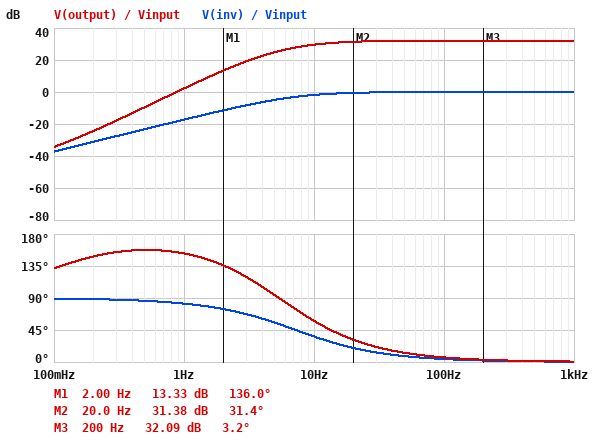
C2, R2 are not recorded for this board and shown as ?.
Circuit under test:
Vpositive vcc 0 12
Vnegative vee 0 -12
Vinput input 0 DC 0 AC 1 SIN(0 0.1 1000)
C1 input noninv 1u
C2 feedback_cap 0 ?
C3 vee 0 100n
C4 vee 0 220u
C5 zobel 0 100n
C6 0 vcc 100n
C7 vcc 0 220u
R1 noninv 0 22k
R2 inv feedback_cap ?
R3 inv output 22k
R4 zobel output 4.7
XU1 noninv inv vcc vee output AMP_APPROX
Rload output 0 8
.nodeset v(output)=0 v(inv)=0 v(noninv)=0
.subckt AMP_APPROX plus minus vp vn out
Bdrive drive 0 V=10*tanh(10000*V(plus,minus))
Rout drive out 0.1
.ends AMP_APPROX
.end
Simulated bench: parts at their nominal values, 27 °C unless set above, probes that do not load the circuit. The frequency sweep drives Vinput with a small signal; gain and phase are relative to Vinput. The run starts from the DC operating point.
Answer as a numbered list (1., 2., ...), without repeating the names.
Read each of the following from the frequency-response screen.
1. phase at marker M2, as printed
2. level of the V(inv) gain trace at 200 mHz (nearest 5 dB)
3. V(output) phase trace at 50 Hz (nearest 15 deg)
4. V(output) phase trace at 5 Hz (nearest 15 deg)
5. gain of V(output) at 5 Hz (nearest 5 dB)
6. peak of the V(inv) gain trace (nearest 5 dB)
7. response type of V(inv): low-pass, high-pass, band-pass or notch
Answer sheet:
1. 31.4 deg
2. -30 dB
3. 15 deg
4. 90 deg
5. 25 dB
6. 0 dB
7. high-pass
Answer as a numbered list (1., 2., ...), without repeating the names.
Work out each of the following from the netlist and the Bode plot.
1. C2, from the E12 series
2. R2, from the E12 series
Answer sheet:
1. 68 µF
2. 560 Ω
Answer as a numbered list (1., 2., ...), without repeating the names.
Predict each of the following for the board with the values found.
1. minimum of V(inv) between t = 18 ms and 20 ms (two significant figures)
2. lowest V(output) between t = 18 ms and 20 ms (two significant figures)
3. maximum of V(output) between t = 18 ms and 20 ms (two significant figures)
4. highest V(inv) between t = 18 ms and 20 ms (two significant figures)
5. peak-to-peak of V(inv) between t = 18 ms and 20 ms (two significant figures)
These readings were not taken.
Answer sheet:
1. -100 mV
2. -4.0 V
3. 4.0 V
4. 100 mV
5. 200 mV
